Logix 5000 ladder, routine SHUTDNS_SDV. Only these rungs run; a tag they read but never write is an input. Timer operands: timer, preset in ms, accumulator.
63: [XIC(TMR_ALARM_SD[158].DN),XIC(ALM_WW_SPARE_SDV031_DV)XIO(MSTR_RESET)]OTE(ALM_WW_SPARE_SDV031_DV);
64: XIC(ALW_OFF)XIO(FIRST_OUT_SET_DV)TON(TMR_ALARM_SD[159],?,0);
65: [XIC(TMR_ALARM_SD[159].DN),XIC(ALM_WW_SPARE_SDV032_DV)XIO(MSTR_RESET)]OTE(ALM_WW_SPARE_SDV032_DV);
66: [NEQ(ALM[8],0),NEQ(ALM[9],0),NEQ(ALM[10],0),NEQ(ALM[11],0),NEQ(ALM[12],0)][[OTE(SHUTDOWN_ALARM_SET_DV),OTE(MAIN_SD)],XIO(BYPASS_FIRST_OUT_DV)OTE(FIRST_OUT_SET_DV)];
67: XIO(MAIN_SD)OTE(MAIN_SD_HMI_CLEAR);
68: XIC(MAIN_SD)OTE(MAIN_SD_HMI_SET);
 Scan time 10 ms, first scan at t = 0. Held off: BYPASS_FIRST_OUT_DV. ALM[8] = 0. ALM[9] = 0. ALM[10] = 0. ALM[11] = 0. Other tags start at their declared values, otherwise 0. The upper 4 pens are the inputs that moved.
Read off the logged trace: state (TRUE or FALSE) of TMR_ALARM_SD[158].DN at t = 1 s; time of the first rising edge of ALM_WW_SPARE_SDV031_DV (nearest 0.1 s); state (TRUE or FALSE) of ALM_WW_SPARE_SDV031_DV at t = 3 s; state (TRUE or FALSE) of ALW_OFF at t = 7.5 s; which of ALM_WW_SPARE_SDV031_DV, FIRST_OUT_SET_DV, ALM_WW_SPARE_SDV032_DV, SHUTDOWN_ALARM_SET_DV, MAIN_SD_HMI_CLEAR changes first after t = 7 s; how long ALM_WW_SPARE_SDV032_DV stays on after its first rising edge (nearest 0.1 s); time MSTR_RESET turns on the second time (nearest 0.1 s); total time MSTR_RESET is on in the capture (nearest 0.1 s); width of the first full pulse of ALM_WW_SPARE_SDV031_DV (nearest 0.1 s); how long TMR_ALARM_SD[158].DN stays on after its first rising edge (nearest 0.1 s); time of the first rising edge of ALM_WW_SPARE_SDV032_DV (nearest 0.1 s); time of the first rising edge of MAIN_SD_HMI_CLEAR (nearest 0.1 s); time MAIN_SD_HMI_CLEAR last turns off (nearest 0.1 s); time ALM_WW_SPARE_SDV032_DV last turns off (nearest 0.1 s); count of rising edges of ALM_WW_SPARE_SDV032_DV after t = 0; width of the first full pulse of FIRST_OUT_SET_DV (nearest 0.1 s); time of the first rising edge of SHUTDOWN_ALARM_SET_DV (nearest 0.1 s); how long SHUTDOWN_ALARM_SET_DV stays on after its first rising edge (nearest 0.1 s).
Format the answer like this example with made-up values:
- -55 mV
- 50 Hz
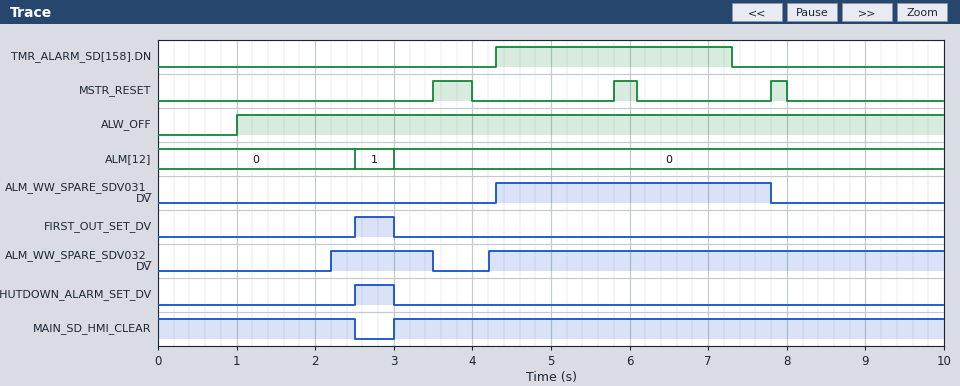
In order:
- FALSE
- 4.3 s
- FALSE
- TRUE
- ALM_WW_SPARE_SDV031_DV
- 1.3 s
- 5.8 s
- 1.0 s
- 3.5 s
- 3.0 s
- 2.2 s
- 3.0 s
- 2.5 s
- 3.5 s
- 2
- 0.5 s
- 2.5 s
- 0.5 s
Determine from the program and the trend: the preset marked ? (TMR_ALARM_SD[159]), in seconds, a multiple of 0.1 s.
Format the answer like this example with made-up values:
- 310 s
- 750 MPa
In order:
- 1.2 s
